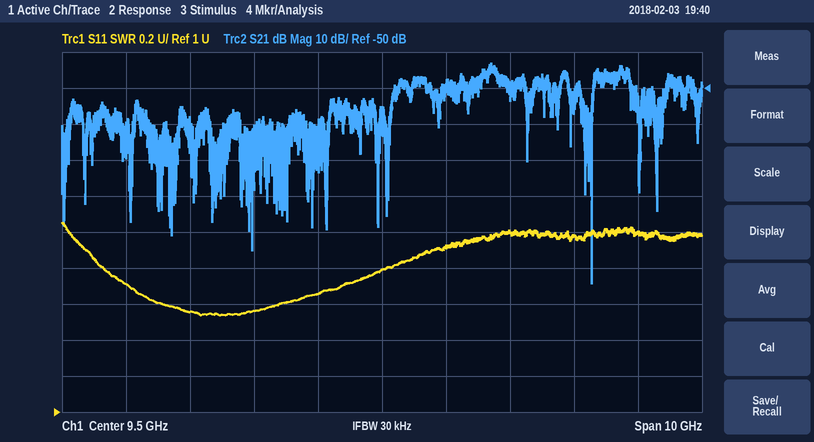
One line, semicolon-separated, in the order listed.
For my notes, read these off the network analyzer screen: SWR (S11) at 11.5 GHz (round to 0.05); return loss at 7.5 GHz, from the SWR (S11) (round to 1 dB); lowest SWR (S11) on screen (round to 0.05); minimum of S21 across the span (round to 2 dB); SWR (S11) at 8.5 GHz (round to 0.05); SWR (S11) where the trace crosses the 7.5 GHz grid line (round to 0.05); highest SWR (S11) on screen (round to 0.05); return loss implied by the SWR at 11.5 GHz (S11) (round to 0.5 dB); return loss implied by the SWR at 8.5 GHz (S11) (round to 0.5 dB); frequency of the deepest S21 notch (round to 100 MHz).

2.00; 13 dB; 1.55; -104 dB; 1.65; 1.55; 2.05; 9.5 dB; 12.0 dB; 12.8 GHz
